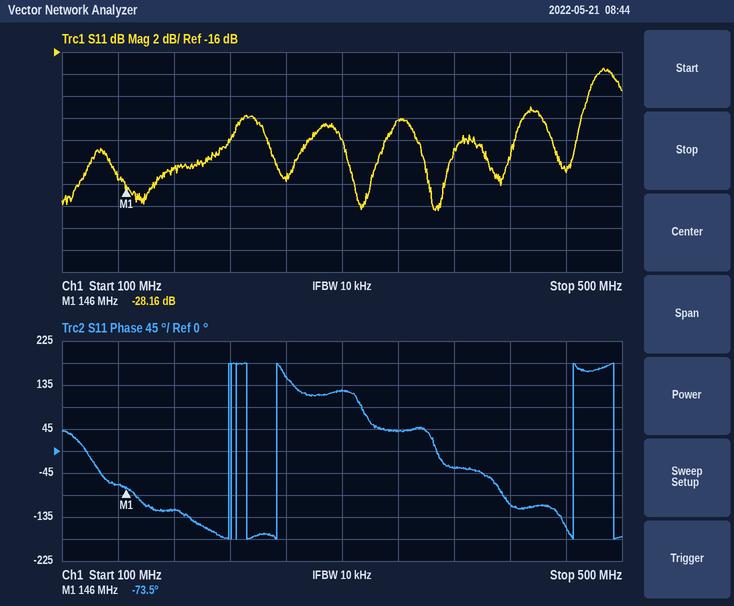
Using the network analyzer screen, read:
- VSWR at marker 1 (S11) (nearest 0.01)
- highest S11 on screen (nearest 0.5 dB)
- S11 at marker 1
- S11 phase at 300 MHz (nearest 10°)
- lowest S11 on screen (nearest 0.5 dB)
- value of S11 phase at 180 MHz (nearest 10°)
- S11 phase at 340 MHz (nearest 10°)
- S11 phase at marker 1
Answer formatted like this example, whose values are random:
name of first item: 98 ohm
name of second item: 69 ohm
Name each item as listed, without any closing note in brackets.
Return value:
VSWR at marker 1 (S11): 1.08
highest S11 on screen: -17.5 dB
S11 at marker 1: -28.16 dB
S11 phase at 300 MHz: 120°
lowest S11 on screen: -30.5 dB
value of S11 phase at 180 MHz: -120°
S11 phase at 340 MHz: 40°
S11 phase at marker 1: -73.5°
